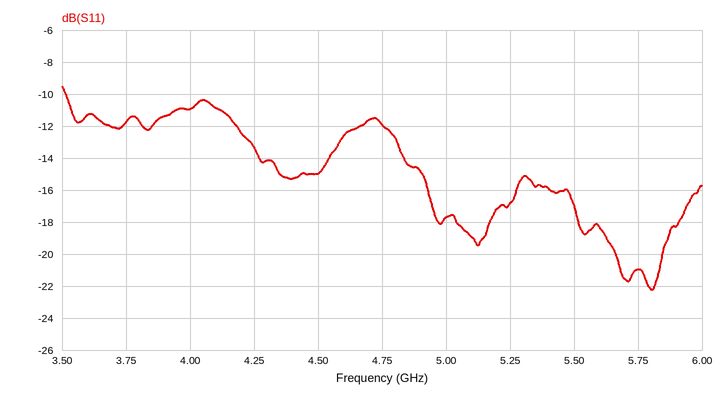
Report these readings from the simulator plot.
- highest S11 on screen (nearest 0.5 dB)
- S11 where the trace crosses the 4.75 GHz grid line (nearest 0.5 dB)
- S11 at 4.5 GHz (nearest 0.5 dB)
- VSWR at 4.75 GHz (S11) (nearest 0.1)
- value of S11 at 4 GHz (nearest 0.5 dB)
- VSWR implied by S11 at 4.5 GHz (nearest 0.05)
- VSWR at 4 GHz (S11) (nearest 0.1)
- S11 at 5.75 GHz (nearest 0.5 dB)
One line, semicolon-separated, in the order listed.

-9.5 dB; -12.0 dB; -15.0 dB; 1.7; -11.0 dB; 1.45; 1.8; -21.0 dB
